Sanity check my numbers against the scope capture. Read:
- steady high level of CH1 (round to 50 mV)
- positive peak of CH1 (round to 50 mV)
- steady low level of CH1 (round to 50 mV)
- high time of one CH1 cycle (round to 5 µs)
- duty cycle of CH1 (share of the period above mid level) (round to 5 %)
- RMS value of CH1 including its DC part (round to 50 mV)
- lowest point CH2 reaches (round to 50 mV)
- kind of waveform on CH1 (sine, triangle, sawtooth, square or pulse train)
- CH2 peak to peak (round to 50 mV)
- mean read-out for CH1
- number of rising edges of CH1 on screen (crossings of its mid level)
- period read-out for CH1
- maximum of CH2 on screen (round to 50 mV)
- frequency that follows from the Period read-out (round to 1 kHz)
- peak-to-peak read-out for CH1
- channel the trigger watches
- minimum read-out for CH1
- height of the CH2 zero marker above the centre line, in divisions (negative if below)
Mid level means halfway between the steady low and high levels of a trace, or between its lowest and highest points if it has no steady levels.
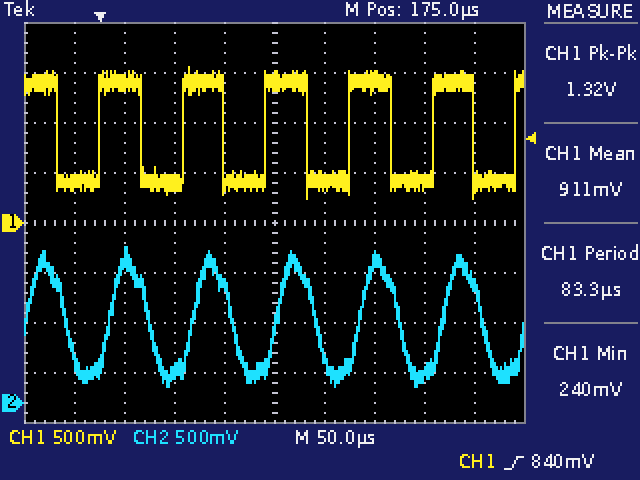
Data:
1.40 V
1.55 V
400 mV
40 µs
50 %
1.05 V
150 mV
square
1.40 V
911 mV
6
83.3 µs
1.55 V
12 kHz
1.32 V
CH1
240 mV
-3.6 div
